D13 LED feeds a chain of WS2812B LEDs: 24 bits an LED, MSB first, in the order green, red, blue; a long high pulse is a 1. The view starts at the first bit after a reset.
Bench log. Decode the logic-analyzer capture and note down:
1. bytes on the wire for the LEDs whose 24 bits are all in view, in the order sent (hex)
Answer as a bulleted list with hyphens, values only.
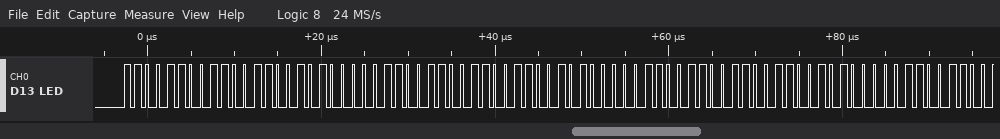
- CC CC A0 CC CC A0 CC CC A0
